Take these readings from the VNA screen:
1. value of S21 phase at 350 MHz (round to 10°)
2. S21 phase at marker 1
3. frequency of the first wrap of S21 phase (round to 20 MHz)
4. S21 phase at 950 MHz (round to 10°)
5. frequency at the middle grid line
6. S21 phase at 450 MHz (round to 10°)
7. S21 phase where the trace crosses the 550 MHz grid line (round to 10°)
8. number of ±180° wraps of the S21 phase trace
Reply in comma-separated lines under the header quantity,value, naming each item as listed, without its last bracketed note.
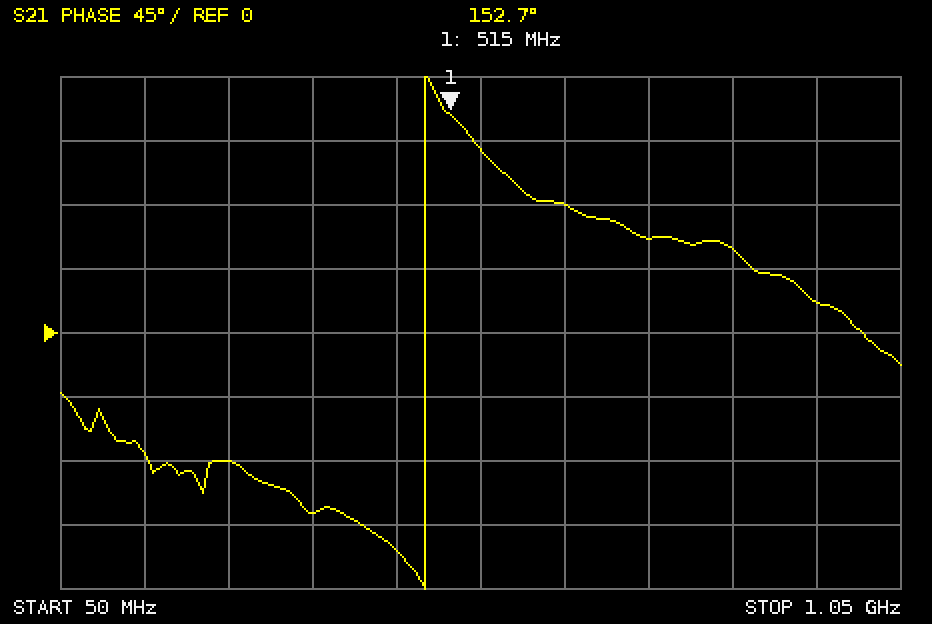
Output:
quantity,value
value of S21 phase at 350 MHz,-130°
S21 phase at marker 1,152.7°
frequency of the first wrap of S21 phase,480 MHz
S21 phase at 950 MHz,20°
frequency at the middle grid line,550 MHz
S21 phase at 450 MHz,-150°
S21 phase where the trace crosses the 550 MHz grid line,130°
number of ±180° wraps of the S21 phase trace,1
